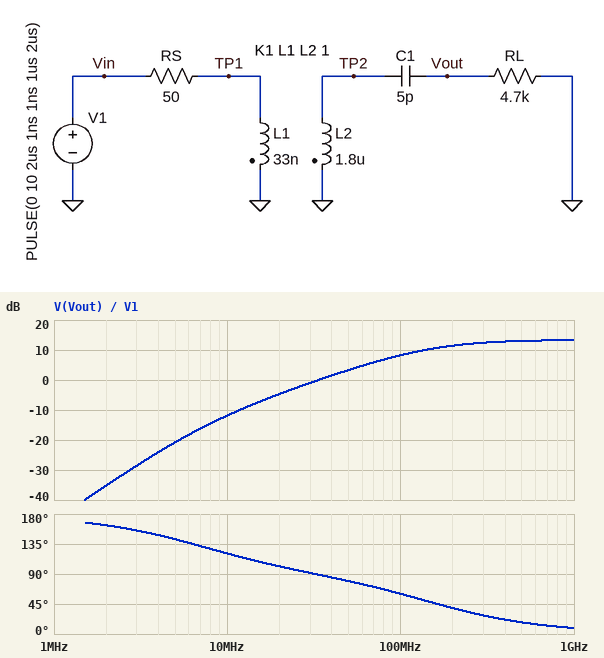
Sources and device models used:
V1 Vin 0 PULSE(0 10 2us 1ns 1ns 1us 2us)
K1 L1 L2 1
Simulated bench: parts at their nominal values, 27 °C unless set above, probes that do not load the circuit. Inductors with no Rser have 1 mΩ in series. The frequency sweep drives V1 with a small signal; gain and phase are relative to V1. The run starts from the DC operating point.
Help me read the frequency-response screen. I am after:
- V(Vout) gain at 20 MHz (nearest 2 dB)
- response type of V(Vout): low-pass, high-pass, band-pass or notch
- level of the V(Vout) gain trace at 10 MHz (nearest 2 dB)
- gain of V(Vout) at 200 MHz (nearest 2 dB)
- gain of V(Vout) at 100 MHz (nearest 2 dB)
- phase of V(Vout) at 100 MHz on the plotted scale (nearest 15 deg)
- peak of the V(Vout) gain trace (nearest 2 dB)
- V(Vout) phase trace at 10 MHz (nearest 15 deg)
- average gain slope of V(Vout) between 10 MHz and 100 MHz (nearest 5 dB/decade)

-4 dB
high-pass
-12 dB
12 dB
8 dB
60 deg
14 dB
120 deg
20 dB/decade
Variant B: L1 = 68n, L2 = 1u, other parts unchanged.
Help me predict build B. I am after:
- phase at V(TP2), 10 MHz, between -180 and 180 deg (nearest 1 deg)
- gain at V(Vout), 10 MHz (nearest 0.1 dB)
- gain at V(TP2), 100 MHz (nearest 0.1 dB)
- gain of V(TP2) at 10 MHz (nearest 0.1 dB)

85 deg
-11.3 dB
7.4 dB
-9.7 dB
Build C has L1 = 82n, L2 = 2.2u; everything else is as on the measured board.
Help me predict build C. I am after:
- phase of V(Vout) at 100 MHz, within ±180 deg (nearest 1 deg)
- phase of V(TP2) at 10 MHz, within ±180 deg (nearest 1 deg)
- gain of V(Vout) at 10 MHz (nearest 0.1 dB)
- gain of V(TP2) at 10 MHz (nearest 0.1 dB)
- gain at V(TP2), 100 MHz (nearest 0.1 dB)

40 deg
83 deg
-7.0 dB
-5.4 dB
10.2 dB
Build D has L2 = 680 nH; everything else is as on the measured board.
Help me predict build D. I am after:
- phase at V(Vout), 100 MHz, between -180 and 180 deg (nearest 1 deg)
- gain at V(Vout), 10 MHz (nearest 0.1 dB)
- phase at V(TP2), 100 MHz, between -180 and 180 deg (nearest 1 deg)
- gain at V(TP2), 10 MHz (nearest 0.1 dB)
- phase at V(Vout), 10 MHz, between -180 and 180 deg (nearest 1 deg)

67 deg
-16.1 dB
63 deg
-14.5 dB
121 deg
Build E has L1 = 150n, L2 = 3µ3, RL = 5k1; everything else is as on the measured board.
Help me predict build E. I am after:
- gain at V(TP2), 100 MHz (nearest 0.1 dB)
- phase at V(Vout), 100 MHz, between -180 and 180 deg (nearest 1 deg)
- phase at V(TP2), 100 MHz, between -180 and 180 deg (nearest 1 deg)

11.0 dB
27 deg
23 deg
